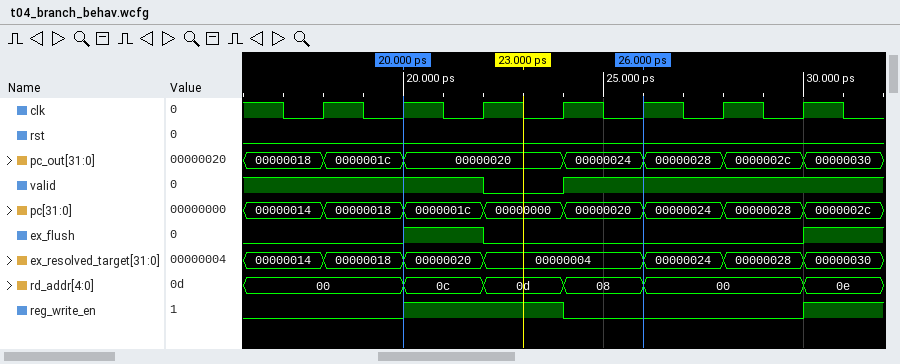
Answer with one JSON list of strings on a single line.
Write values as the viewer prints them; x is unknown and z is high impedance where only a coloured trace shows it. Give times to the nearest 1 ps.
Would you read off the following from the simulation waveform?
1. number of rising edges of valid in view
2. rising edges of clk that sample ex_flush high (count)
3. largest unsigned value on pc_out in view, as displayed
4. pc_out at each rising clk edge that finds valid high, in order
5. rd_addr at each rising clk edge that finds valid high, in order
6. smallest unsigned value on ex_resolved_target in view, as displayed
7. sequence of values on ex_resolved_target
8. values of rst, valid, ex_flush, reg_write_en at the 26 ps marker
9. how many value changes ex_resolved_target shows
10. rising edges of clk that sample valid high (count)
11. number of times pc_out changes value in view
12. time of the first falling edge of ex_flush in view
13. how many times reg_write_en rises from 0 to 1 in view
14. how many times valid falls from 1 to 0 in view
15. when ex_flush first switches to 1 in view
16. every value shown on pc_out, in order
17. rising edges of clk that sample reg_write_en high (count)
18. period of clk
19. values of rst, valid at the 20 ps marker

["1", "1", "00000030", "00000018, 0000001c, 00000020, 00000024, 00000028, 0000002c", "00, 00, 0c, 08, 00, 00", "00000004", "00000014, 00000018, 00000020, 00000004, 00000024, 00000028, 00000030", "rst=0, valid=1, ex_flush=0, reg_write_en=0", "6", "6", "6", "22 ps", "2", "1", "20 ps", "00000018, 0000001c, 00000020, 00000024, 00000028, 0000002c, 00000030", "2", "2 ps", "rst=0, valid=1"]
